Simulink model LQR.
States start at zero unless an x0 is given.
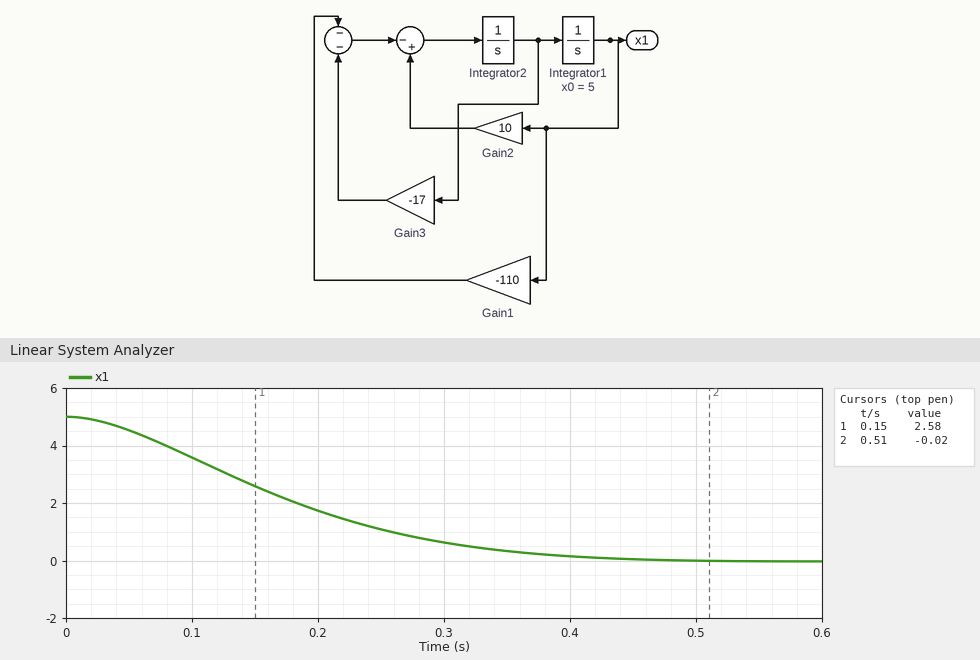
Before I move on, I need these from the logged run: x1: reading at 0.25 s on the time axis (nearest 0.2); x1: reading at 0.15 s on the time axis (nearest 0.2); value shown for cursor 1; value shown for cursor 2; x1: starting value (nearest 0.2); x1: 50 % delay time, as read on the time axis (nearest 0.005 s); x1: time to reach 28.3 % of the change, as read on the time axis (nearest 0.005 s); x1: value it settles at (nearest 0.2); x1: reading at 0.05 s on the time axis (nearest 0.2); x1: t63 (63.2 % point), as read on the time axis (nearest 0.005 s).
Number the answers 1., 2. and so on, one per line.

1. 1.0
2. 2.6
3. 2.58
4. -0.02
5. 5.0
6. 0.155 s
7. 0.100 s
8. 0.0
9. 4.6
10. 0.195 s
